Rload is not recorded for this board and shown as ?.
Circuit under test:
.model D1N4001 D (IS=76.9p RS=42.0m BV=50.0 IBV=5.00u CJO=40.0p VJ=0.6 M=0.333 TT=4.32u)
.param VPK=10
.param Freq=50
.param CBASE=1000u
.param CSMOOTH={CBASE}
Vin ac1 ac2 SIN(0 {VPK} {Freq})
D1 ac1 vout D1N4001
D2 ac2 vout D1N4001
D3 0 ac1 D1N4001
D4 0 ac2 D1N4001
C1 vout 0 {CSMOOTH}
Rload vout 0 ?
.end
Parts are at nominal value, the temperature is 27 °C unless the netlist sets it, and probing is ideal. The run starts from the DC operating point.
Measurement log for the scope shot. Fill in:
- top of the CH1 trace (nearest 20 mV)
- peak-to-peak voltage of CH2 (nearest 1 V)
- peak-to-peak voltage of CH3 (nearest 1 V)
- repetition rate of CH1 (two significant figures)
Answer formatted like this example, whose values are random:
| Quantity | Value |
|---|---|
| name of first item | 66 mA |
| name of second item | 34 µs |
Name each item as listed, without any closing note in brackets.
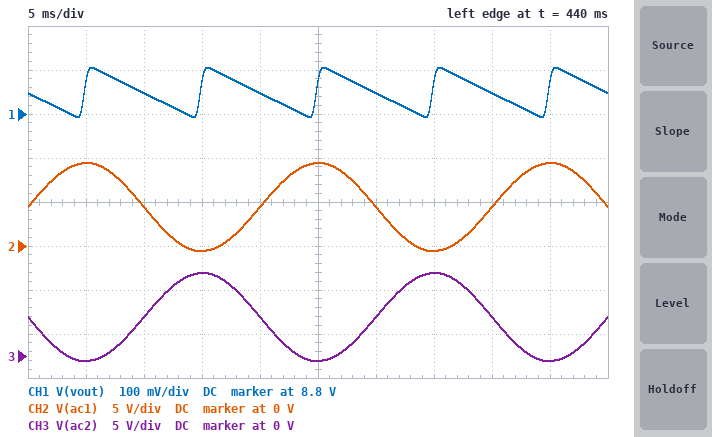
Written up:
| Quantity | Value |
|---|---|
| top of the CH1 trace | 8.90 V |
| peak-to-peak voltage of CH2 | 10 V |
| peak-to-peak voltage of CH3 | 10 V |
| repetition rate of CH1 | 100 Hz |
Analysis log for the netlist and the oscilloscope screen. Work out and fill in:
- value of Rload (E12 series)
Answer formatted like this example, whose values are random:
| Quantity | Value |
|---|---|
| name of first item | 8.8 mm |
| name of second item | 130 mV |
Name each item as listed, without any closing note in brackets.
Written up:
| Quantity | Value |
|---|---|
| value of Rload | 680 Ω |
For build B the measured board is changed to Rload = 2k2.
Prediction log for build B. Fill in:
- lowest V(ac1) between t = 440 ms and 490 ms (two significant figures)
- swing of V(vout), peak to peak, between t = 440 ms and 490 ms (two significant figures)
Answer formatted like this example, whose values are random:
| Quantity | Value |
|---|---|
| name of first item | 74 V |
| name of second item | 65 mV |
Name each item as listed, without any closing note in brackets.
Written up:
| Quantity | Value |
|---|---|
| lowest V(ac1) between t = 440 ms and 490 ms | -540 mV |
| swing of V(vout), peak to peak, between t = 440 ms and 490 ms | 35 mV |
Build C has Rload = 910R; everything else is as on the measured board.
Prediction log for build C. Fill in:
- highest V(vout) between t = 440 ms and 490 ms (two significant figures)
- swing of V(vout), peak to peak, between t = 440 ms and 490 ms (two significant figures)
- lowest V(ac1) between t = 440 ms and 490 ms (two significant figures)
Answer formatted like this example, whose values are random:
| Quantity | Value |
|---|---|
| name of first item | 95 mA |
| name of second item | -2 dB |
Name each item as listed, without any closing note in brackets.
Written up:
| Quantity | Value |
|---|---|
| highest V(vout) between t = 440 ms and 490 ms | 8.9 V |
| swing of V(vout), peak to peak, between t = 440 ms and 490 ms | 85 mV |
| lowest V(ac1) between t = 440 ms and 490 ms | -560 mV |
